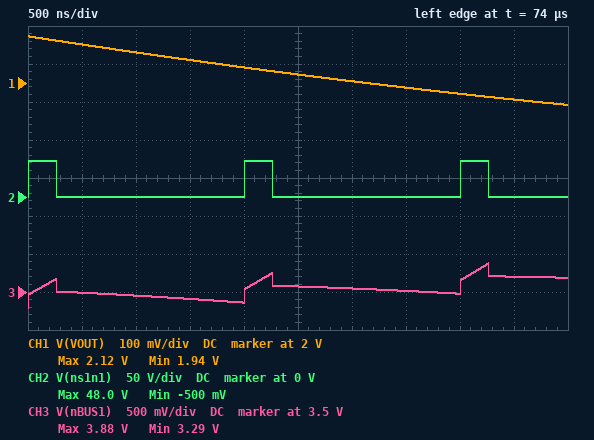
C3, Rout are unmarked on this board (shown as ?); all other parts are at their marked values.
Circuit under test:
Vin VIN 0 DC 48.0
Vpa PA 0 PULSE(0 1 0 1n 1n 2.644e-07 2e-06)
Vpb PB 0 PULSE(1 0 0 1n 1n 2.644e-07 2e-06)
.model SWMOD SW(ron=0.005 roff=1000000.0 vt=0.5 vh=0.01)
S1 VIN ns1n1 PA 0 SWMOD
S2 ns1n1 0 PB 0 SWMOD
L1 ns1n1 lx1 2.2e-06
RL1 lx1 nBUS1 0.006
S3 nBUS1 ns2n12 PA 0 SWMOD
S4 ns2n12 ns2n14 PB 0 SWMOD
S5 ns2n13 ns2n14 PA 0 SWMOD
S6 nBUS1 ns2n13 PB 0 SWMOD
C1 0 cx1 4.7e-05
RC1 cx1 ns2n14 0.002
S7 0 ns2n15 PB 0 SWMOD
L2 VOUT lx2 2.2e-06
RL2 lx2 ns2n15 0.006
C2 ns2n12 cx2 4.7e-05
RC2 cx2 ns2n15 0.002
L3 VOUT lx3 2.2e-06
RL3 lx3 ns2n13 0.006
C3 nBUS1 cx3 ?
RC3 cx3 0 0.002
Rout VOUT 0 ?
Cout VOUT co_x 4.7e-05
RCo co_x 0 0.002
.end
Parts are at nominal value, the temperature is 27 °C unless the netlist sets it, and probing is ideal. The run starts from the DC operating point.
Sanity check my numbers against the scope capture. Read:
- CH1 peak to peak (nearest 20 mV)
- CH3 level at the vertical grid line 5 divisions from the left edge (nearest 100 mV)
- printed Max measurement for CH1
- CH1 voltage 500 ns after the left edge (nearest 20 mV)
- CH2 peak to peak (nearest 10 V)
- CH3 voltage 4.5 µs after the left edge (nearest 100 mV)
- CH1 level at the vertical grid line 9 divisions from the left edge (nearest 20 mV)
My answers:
180 mV
3.6 V
2.12 V
2.10 V
50 V
3.7 V
1.96 V
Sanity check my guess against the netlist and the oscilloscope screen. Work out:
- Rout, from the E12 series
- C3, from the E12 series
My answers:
0.068 Ω
100 µF
